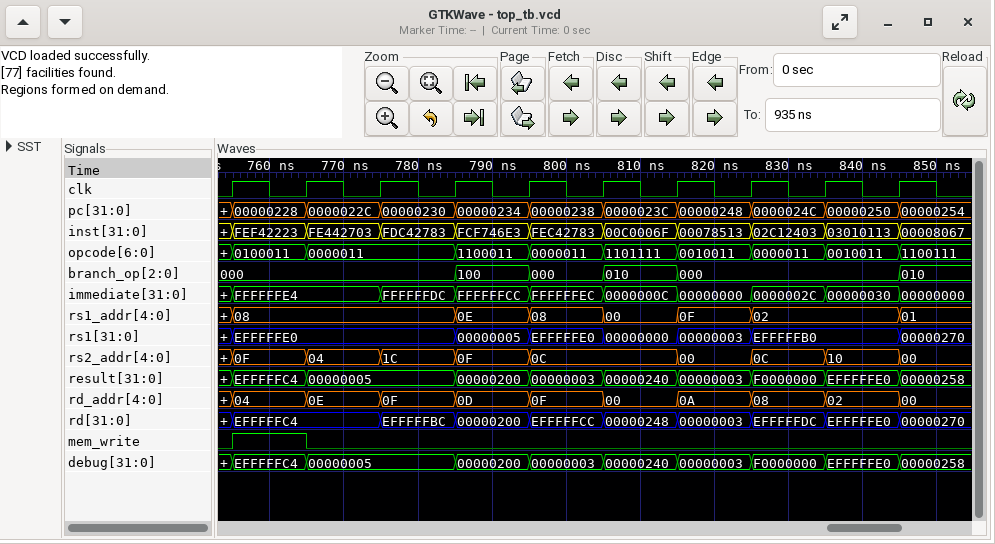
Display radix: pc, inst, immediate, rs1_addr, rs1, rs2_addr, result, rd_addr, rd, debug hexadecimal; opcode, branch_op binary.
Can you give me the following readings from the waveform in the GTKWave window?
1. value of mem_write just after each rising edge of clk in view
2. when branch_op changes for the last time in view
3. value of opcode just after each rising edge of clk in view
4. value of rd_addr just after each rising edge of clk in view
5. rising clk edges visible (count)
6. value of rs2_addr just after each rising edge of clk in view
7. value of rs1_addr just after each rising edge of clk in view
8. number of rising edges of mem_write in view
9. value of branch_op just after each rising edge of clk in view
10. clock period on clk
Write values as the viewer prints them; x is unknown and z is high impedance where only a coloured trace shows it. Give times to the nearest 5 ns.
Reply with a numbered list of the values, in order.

1. 1 0 0 0 0 0 0 0 0 0
2. 845 ns
3. 0100011, 0000011, 0000011, 1100011, 0000011, 1101111, 0010011, 0000011, 0010011, 1100111
4. 04, 0E, 0F, 0D, 0F, 00, 0A, 08, 02, 00
5. 10
6. 0F, 04, 1C, 0F, 0C, 0C, 00, 0C, 10, 00
7. 08, 08, 08, 0E, 08, 00, 0F, 02, 02, 01
8. 1
9. 000, 000, 000, 100, 000, 010, 000, 000, 000, 010
10. 10 ns
